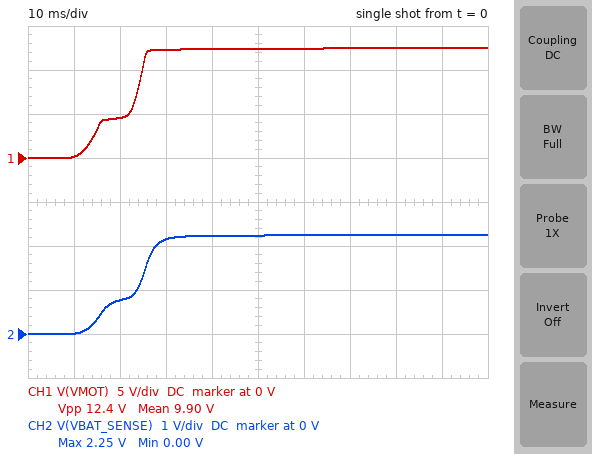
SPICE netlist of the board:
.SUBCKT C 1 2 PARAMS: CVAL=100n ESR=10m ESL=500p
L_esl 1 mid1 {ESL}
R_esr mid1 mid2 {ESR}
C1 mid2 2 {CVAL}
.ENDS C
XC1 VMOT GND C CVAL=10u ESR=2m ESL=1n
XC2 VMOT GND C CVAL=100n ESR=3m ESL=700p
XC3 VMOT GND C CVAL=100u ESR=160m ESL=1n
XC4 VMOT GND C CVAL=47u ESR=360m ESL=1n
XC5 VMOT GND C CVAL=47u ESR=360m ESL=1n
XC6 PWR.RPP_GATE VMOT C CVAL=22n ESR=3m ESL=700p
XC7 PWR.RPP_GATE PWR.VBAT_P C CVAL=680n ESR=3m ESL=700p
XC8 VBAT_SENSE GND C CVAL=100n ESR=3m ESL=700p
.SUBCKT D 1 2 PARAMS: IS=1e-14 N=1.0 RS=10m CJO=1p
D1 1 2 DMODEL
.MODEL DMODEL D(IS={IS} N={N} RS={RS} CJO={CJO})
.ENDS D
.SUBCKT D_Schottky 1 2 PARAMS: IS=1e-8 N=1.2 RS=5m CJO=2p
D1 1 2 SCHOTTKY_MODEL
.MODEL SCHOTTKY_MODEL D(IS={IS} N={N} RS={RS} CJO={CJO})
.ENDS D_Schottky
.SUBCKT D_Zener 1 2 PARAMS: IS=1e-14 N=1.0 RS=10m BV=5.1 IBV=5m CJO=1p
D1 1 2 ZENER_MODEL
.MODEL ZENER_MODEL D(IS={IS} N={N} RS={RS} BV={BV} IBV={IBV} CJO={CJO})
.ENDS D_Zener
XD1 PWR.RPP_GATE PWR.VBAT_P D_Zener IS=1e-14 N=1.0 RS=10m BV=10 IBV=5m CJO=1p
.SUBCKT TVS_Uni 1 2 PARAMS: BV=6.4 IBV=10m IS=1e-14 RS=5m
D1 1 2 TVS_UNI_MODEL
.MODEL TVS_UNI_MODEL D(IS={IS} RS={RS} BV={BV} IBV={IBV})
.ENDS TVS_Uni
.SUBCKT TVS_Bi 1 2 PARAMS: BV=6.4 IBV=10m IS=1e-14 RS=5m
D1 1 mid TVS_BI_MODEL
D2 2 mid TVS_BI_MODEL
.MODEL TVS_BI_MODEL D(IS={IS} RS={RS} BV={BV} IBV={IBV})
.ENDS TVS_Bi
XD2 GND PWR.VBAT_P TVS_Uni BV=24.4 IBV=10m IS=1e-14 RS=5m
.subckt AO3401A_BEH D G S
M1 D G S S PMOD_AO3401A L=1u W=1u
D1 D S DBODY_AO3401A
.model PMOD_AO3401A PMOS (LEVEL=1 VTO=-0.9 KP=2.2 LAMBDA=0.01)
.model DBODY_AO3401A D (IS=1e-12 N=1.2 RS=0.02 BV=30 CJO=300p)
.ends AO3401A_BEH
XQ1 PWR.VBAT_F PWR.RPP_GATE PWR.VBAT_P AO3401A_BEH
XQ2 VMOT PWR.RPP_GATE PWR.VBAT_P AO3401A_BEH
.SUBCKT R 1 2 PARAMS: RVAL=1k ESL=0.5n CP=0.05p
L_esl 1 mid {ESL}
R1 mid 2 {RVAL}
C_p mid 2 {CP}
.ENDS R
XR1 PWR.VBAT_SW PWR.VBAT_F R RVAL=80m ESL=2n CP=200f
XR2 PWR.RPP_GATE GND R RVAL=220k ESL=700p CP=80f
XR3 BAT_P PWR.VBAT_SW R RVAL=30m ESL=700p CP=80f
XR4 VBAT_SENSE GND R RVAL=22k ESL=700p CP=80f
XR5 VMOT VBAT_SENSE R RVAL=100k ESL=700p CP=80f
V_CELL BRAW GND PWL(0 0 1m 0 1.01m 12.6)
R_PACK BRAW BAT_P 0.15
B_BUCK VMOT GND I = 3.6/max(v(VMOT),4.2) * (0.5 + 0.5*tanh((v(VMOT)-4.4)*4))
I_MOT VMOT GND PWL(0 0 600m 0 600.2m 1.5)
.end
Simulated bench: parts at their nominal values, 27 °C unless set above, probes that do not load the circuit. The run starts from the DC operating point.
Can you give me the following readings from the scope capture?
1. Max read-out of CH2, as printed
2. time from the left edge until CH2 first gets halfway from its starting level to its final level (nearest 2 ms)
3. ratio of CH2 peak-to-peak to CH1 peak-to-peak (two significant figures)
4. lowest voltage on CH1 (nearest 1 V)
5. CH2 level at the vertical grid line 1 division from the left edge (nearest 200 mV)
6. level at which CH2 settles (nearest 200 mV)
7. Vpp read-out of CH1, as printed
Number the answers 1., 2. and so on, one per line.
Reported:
1. 2.25 V
2. 24 ms
3. 0.18
4. 0 V
5. 0 V
6. 2.2 V
7. 12.4 V
